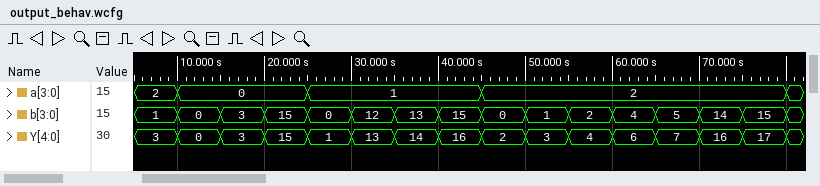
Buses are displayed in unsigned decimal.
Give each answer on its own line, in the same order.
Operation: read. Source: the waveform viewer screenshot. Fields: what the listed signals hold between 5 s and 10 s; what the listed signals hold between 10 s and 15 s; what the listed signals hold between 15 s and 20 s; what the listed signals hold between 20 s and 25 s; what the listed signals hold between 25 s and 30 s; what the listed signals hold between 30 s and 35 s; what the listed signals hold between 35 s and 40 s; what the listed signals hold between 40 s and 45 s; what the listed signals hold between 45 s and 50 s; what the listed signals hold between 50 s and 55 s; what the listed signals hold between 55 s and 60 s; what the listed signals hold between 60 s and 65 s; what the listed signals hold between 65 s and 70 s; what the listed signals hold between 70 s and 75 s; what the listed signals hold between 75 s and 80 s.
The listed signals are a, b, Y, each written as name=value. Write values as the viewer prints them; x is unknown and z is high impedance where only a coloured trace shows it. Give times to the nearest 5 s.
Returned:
a=2, b=1, Y=3
a=0, b=0, Y=0
a=0, b=3, Y=3
a=0, b=15, Y=15
a=1, b=0, Y=1
a=1, b=12, Y=13
a=1, b=13, Y=14
a=1, b=15, Y=16
a=2, b=0, Y=2
a=2, b=1, Y=3
a=2, b=2, Y=4
a=2, b=4, Y=6
a=2, b=5, Y=7
a=2, b=14, Y=16
a=2, b=15, Y=17
